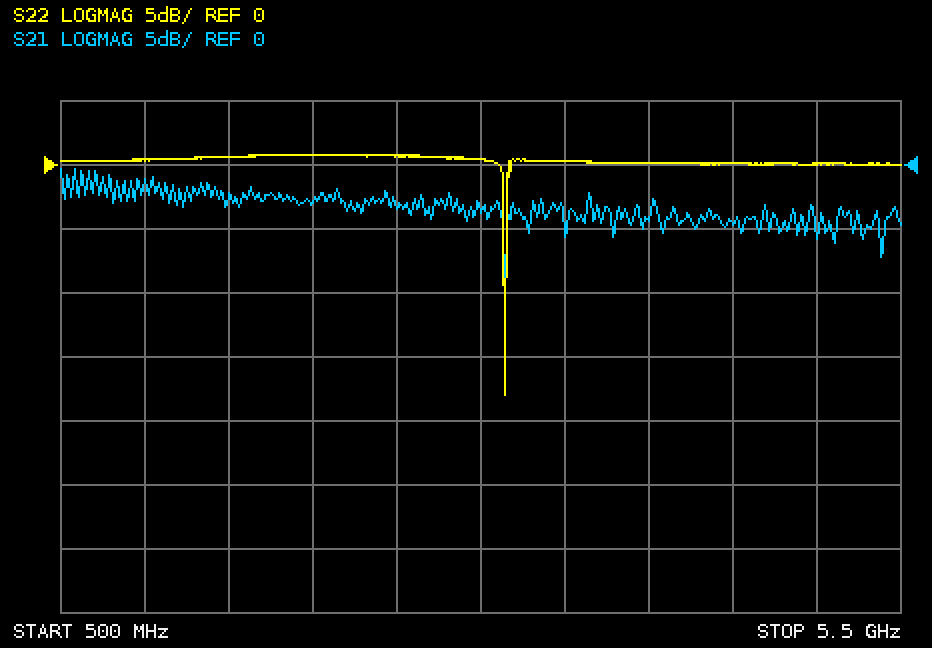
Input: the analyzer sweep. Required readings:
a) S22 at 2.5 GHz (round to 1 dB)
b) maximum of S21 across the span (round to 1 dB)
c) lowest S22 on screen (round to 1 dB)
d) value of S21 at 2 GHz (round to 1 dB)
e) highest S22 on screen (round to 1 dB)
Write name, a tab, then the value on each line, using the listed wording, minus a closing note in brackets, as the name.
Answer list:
S22 at 2.5 GHz	1 dB
maximum of S21 across the span	0 dB
lowest S22 on screen	-18 dB
value of S21 at 2 GHz	-3 dB
highest S22 on screen	1 dB
